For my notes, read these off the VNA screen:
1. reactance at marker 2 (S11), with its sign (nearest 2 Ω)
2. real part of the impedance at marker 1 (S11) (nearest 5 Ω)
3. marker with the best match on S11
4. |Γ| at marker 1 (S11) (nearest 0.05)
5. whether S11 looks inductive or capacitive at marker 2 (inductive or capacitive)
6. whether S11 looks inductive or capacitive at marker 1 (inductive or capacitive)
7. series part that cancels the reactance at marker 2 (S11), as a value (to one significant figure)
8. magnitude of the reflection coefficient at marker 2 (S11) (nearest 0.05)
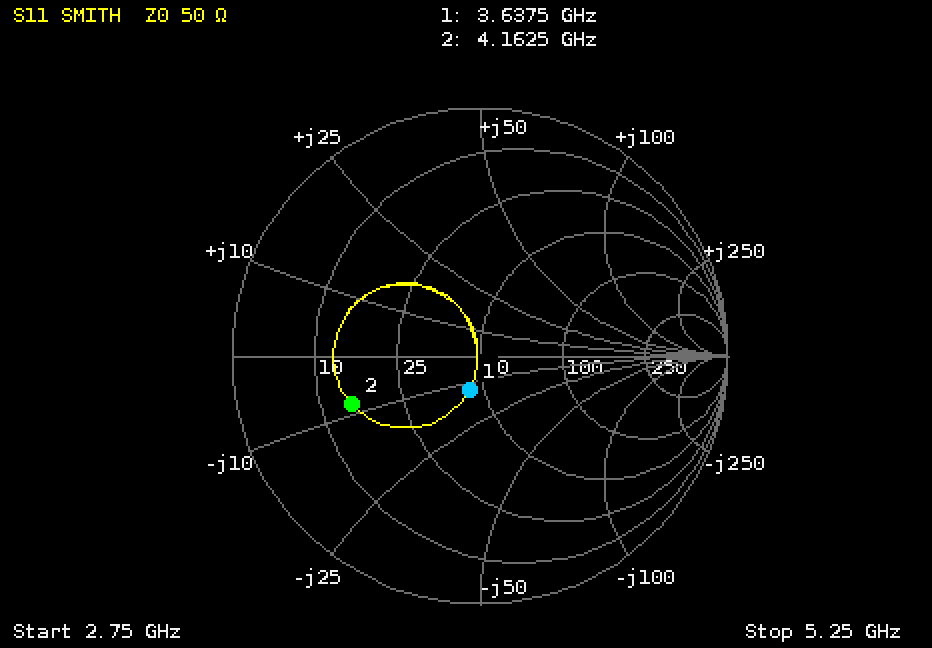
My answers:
-8 Ω
45 Ω
marker 1
0.15
capacitive
capacitive
300 pH
0.55
